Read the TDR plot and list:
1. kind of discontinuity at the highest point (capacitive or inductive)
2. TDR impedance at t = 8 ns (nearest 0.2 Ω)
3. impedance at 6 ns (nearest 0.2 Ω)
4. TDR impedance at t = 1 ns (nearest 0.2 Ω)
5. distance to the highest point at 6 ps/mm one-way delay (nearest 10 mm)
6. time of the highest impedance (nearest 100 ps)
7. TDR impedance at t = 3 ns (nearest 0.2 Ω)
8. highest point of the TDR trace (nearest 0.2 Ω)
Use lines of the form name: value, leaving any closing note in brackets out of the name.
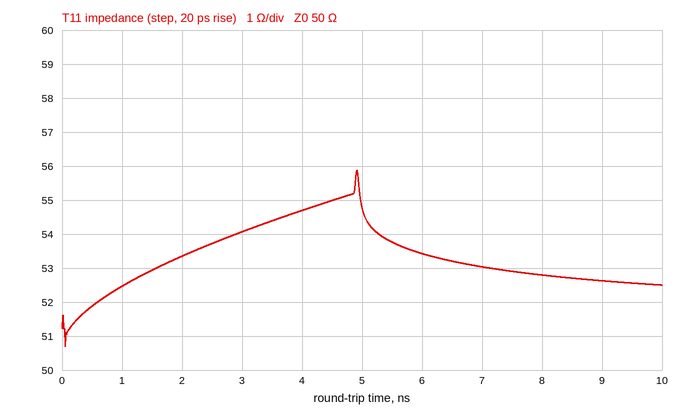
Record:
kind of discontinuity at the highest point: inductive
TDR impedance at t = 8 ns: 52.8 Ω
impedance at 6 ns: 53.4 Ω
TDR impedance at t = 1 ns: 52.4 Ω
distance to the highest point at 6 ps/mm one-way delay: 410 mm
time of the highest impedance: 4.9 ns
TDR impedance at t = 3 ns: 54.0 Ω
highest point of the TDR trace: 55.8 Ω
